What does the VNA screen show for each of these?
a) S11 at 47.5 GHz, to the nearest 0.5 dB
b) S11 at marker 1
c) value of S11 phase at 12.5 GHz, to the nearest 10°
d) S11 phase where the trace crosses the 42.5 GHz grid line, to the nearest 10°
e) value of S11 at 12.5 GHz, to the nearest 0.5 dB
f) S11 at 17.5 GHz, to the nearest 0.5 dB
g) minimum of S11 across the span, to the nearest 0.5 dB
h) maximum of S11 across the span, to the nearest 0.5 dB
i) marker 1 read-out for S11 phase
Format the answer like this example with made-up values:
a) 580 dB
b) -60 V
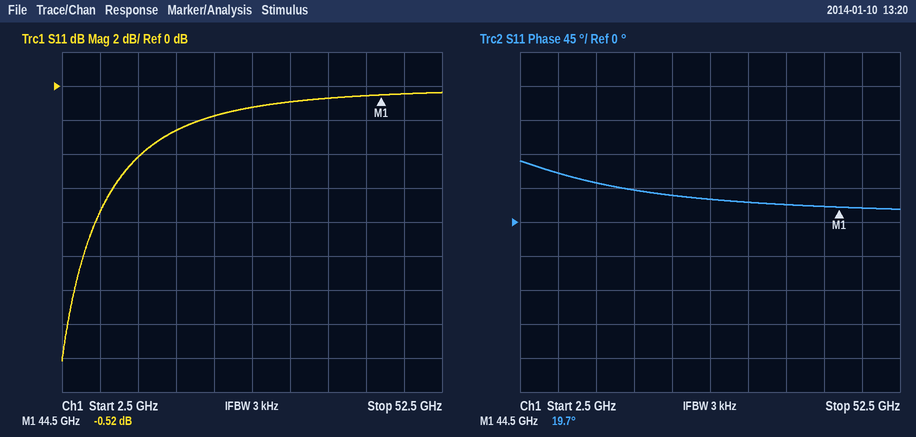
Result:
a) -0.5 dB
b) -0.52 dB
c) 50°
d) 20°
e) -4.0 dB
f) -2.5 dB
g) -16.0 dB
h) -0.5 dB
i) 19.7°
